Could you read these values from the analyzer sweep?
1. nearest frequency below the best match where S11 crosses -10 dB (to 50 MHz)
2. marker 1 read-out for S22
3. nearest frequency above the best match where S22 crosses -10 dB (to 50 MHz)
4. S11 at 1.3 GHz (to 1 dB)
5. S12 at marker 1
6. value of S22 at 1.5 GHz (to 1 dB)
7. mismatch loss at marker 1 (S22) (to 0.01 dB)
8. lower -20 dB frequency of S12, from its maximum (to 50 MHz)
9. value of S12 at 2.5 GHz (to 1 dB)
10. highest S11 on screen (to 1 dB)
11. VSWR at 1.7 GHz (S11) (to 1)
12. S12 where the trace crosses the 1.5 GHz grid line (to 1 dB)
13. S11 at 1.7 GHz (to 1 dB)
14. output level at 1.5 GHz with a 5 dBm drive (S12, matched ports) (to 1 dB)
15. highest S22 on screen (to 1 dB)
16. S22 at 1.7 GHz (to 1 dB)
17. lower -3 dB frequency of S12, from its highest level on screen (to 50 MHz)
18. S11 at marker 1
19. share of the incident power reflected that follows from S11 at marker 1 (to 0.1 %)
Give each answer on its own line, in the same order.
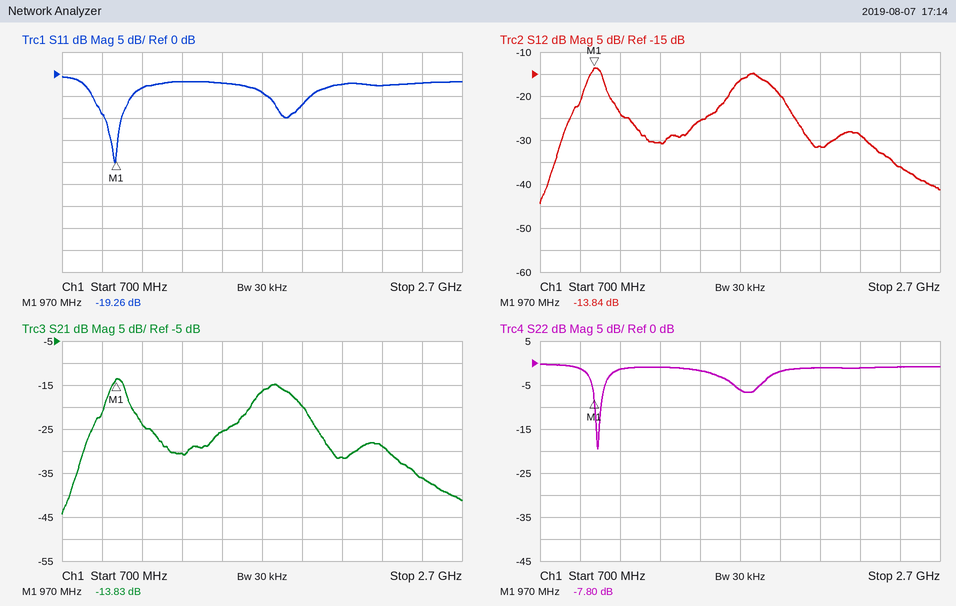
900 MHz
-7.80 dB
1.00 GHz
-2 dB
-13.84 dB
-2 dB
0.79 dB
800 MHz
-36 dB
-1 dB
4
-26 dB
-4 dB
-21 dBm
0 dB
-6 dB
950 MHz
-19.26 dB
1.2 %
